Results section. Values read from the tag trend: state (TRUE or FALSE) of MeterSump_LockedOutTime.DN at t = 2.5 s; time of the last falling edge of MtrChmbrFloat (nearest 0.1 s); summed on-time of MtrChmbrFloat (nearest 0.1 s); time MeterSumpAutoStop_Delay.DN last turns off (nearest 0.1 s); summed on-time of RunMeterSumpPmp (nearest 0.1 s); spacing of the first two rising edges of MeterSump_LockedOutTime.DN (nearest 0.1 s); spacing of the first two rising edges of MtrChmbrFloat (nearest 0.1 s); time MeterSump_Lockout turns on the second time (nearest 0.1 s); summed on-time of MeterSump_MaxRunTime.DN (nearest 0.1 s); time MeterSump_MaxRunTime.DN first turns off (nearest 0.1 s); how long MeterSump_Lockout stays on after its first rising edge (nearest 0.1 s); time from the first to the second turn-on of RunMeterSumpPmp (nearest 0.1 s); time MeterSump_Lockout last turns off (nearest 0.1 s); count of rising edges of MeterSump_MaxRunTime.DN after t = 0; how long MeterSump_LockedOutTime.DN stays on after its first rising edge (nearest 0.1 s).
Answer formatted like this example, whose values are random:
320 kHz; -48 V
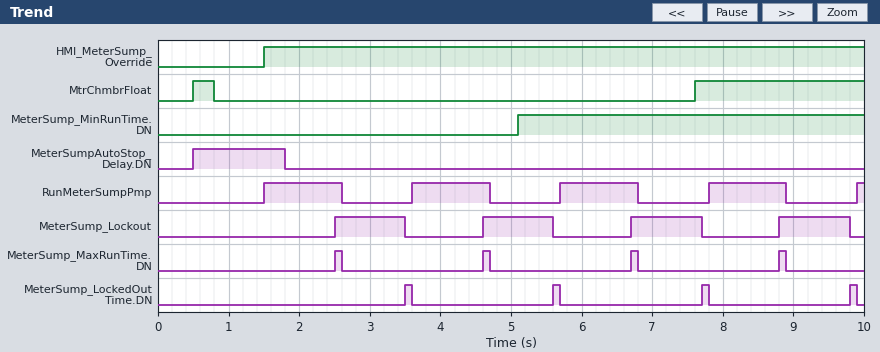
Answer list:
FALSE; 0.8 s; 2.7 s; 1.8 s; 4.5 s; 2.1 s; 7.1 s; 4.6 s; 0.4 s; 2.6 s; 1.0 s; 2.1 s; 9.8 s; 4; 0.1 s
